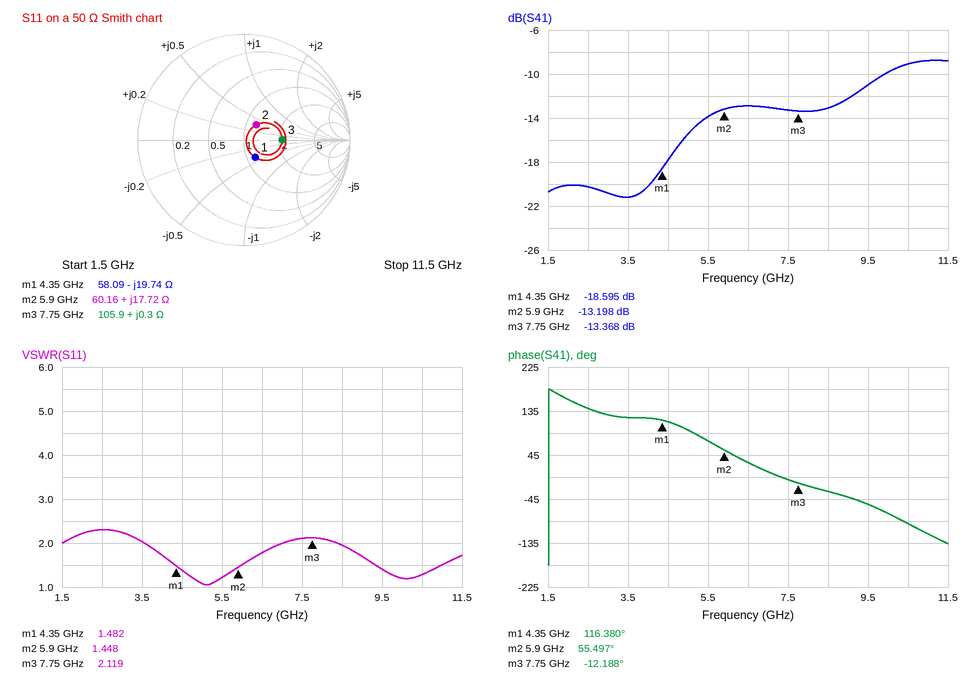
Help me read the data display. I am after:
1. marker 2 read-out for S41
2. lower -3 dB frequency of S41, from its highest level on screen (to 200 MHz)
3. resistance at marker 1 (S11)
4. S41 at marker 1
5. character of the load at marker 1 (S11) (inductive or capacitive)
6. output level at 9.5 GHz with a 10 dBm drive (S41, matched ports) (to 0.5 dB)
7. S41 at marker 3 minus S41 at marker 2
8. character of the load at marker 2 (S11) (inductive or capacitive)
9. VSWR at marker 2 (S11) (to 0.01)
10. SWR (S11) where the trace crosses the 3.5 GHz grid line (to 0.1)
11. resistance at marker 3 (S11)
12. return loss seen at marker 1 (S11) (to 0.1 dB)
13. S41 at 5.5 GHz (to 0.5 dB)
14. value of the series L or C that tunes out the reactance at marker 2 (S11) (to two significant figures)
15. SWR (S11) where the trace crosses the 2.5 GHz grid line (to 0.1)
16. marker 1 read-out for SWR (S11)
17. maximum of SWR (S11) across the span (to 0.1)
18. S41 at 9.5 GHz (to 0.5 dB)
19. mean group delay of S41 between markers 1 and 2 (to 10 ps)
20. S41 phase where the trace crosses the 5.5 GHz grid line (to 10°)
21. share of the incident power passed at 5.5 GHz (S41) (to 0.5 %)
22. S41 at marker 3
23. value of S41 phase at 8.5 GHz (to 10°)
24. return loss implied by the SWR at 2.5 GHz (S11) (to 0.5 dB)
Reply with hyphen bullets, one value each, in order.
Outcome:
- -13.198 dB
- 9.2 GHz
- 58.09 Ω
- -18.595 dB
- capacitive
- -1.0 dBm
- -0.170 dB
- inductive
- 1.45
- 2.0
- 105.9 Ω
- 14.2 dB
- -14.0 dB
- 1.5 pF
- 2.3
- 1.482
- 2.3
- -11.0 dB
- 110 ps
- 70°
- 4.0 %
- -13.368 dB
- -30°
- 8.0 dB
